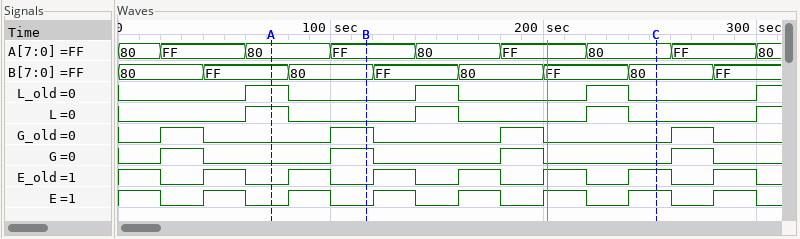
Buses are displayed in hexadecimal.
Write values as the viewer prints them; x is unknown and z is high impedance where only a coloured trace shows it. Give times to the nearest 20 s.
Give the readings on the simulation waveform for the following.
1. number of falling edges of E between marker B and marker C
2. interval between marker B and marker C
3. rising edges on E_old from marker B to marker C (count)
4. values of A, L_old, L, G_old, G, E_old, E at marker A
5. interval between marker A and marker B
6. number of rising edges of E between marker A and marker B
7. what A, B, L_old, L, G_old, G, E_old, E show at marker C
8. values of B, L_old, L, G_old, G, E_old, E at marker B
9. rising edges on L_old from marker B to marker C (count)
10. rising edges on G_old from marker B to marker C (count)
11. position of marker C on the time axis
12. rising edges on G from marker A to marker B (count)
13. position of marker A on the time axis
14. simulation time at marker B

3
140 s
4
A=80, L_old=1, L=1, G_old=0, G=0, E_old=0, E=0
40 s
1
A=80, B=80, L_old=0, L=0, G_old=0, G=0, E_old=1, E=1
B=80, L_old=0, L=0, G_old=1, G=1, E_old=0, E=0
2
1
260 s
1
80 s
120 s
